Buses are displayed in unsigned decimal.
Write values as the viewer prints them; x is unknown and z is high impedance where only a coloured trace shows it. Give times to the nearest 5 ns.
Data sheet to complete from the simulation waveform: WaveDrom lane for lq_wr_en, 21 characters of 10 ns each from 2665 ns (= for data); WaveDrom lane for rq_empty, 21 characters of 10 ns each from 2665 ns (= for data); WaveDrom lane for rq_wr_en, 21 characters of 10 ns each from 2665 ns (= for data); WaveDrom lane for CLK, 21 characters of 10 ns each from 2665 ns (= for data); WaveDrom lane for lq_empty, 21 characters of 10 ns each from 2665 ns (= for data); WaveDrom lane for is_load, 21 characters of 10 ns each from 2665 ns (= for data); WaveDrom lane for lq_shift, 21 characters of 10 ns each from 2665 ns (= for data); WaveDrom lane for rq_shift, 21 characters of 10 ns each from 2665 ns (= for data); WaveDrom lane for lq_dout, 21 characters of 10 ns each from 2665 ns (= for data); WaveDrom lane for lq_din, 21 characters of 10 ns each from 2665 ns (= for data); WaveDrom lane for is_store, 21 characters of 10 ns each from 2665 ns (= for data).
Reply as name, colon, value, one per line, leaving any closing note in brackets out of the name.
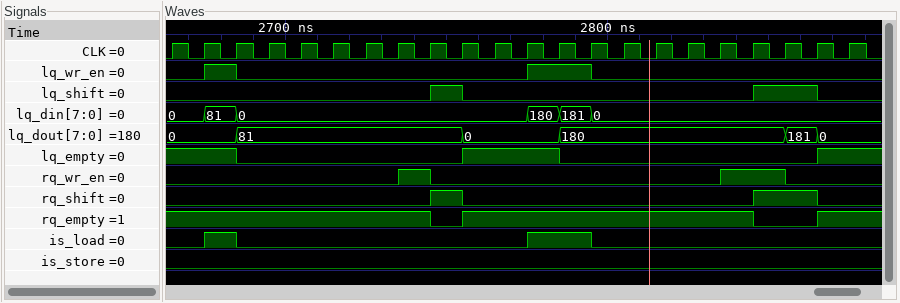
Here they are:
WaveDrom lane for lq_wr_en, 21 characters of 10 ns each from 2665 ns: {name: 'lq_wr_en', wave: '010........1.0.......'}
WaveDrom lane for rq_empty, 21 characters of 10 ns each from 2665 ns: {name: 'rq_empty', wave: '1.......01........0.1'}
WaveDrom lane for rq_wr_en, 21 characters of 10 ns each from 2665 ns: {name: 'rq_wr_en', wave: '0......10........1.0.'}
WaveDrom lane for CLK, 21 characters of 10 ns each from 2665 ns: {name: 'CLK', wave: 'p....................'}
WaveDrom lane for lq_empty, 21 characters of 10 ns each from 2665 ns: {name: 'lq_empty', wave: '1.0......1..0.......1'}
WaveDrom lane for is_load, 21 characters of 10 ns each from 2665 ns: {name: 'is_load', wave: '010........1.0.......'}
WaveDrom lane for lq_shift, 21 characters of 10 ns each from 2665 ns: {name: 'lq_shift', wave: '0.......10........1.0'}
WaveDrom lane for rq_shift, 21 characters of 10 ns each from 2665 ns: {name: 'rq_shift', wave: '0.......10........1.0'}
WaveDrom lane for lq_dout, 21 characters of 10 ns each from 2665 ns: {name: 'lq_dout', wave: '=.=......=..=......==', data: '0 81 0 180 181 0'}
WaveDrom lane for lq_din, 21 characters of 10 ns each from 2665 ns: {name: 'lq_din', wave: '===........===.......', data: '0 81 0 180 181 0'}
WaveDrom lane for is_store, 21 characters of 10 ns each from 2665 ns: {name: 'is_store', wave: '0....................'}
